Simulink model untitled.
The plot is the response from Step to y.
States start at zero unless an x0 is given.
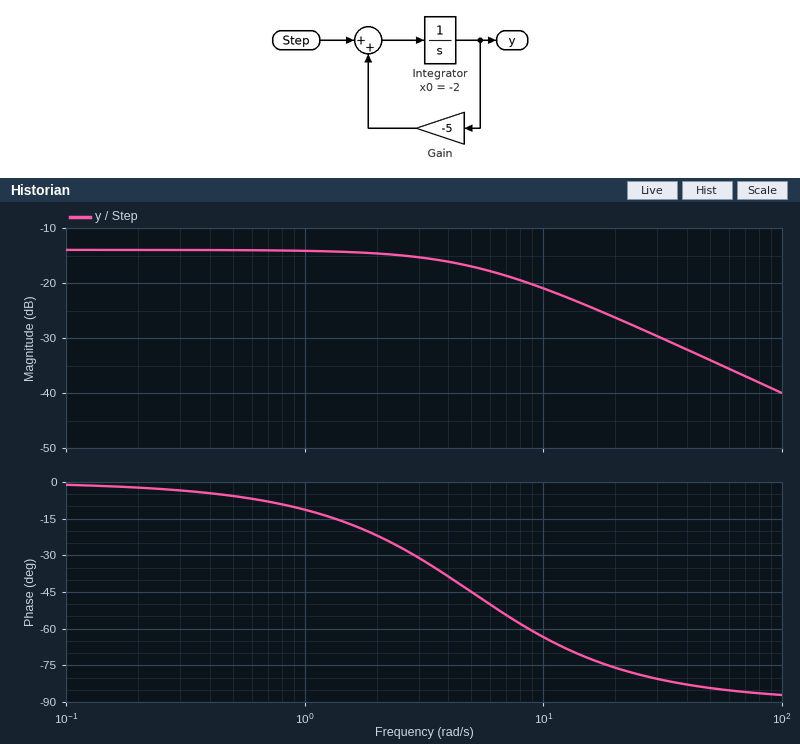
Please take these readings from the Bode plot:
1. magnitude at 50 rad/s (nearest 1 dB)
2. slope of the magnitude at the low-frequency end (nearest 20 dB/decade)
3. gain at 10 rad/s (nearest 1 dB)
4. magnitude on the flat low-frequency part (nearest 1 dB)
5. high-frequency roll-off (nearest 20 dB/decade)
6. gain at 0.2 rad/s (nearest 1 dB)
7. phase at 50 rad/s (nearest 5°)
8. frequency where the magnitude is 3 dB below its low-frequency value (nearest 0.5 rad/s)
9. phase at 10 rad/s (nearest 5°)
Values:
-34 dB
0 dB/decade
-21 dB
-14 dB
-20 dB/decade
-14 dB
-85°
5.0 rad/s
-65°
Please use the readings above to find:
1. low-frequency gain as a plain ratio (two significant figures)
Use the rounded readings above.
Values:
0.20
